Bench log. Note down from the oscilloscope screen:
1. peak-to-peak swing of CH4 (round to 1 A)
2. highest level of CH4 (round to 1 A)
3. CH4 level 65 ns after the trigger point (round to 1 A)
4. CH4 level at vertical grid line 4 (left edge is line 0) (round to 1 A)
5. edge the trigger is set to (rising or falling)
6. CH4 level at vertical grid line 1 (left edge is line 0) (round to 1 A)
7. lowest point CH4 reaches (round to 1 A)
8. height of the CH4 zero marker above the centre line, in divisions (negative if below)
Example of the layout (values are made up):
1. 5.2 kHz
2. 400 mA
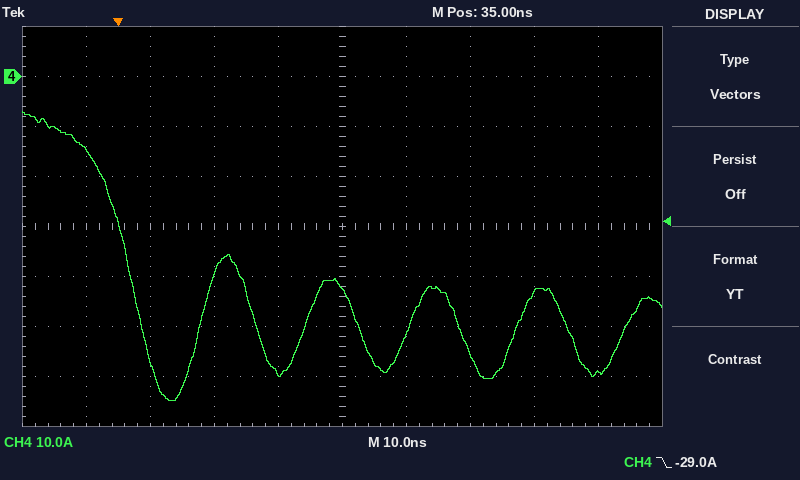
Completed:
1. 58 A
2. -7 A
3. -43 A
4. -59 A
5. falling
6. -15 A
7. -65 A
8. +3.0 div
